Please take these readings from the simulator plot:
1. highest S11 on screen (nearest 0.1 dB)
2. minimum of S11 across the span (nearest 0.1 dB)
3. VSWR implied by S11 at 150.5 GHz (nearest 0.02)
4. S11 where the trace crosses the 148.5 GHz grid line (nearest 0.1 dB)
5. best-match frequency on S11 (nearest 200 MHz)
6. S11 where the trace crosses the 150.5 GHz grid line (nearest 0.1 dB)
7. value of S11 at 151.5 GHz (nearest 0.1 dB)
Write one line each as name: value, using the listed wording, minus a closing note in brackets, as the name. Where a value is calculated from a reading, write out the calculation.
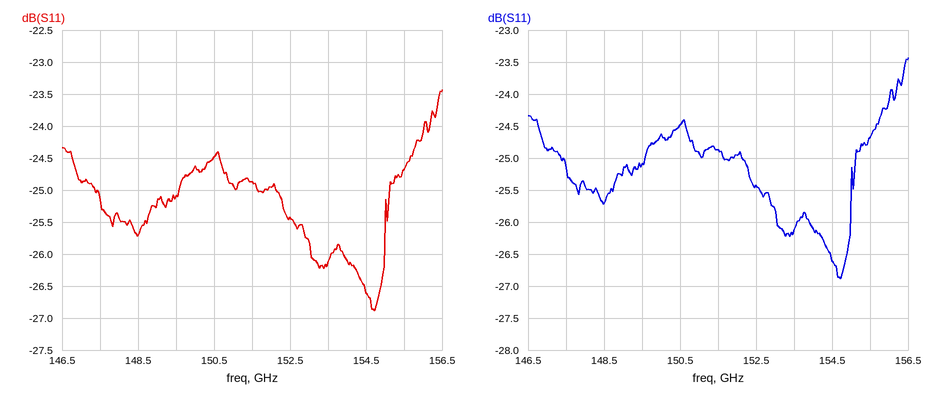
highest S11 on screen: -23.4 dB
minimum of S11 across the span: -26.9 dB
VSWR implied by S11 at 150.5 GHz: |Γ| = 10^(-24.5/20) = 0.0596; VSWR = (1 + 0.0596)/(1 − 0.0596) ≈ 1.13, so 1.12 to the nearest 0.02
S11 where the trace crosses the 148.5 GHz grid line: -25.7 dB
best-match frequency on S11: 154.8 GHz
S11 where the trace crosses the 150.5 GHz grid line: -24.5 dB
value of S11 at 151.5 GHz: -24.9 dB
